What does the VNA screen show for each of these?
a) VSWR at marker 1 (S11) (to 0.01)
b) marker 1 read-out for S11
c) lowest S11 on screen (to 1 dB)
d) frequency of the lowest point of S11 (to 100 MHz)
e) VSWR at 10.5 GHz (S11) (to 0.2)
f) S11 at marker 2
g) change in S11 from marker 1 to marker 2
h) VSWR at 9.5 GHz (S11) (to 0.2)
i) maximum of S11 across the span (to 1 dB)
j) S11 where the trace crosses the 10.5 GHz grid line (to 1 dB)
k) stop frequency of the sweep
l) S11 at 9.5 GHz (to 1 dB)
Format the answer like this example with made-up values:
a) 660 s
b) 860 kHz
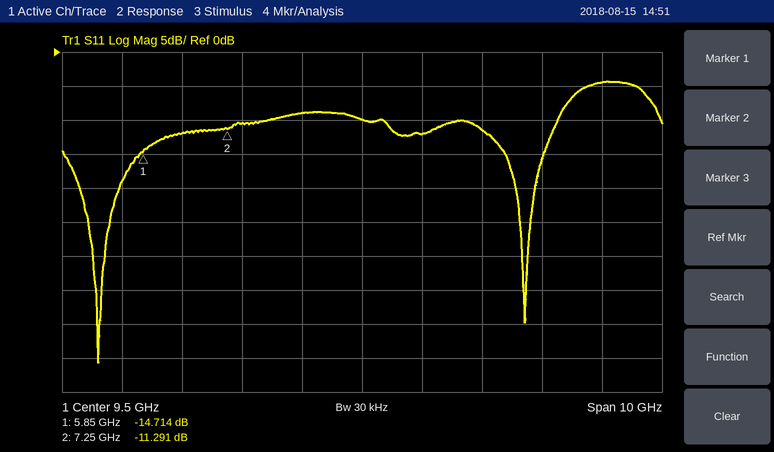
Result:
a) 1.45
b) -14.714 dB
c) -46 dB
d) 5.1 GHz
e) 1.6
f) -11.291 dB
g) 3.423 dB
h) 2.0
i) -4 dB
j) -12 dB
k) 14.5 GHz
l) -10 dB
